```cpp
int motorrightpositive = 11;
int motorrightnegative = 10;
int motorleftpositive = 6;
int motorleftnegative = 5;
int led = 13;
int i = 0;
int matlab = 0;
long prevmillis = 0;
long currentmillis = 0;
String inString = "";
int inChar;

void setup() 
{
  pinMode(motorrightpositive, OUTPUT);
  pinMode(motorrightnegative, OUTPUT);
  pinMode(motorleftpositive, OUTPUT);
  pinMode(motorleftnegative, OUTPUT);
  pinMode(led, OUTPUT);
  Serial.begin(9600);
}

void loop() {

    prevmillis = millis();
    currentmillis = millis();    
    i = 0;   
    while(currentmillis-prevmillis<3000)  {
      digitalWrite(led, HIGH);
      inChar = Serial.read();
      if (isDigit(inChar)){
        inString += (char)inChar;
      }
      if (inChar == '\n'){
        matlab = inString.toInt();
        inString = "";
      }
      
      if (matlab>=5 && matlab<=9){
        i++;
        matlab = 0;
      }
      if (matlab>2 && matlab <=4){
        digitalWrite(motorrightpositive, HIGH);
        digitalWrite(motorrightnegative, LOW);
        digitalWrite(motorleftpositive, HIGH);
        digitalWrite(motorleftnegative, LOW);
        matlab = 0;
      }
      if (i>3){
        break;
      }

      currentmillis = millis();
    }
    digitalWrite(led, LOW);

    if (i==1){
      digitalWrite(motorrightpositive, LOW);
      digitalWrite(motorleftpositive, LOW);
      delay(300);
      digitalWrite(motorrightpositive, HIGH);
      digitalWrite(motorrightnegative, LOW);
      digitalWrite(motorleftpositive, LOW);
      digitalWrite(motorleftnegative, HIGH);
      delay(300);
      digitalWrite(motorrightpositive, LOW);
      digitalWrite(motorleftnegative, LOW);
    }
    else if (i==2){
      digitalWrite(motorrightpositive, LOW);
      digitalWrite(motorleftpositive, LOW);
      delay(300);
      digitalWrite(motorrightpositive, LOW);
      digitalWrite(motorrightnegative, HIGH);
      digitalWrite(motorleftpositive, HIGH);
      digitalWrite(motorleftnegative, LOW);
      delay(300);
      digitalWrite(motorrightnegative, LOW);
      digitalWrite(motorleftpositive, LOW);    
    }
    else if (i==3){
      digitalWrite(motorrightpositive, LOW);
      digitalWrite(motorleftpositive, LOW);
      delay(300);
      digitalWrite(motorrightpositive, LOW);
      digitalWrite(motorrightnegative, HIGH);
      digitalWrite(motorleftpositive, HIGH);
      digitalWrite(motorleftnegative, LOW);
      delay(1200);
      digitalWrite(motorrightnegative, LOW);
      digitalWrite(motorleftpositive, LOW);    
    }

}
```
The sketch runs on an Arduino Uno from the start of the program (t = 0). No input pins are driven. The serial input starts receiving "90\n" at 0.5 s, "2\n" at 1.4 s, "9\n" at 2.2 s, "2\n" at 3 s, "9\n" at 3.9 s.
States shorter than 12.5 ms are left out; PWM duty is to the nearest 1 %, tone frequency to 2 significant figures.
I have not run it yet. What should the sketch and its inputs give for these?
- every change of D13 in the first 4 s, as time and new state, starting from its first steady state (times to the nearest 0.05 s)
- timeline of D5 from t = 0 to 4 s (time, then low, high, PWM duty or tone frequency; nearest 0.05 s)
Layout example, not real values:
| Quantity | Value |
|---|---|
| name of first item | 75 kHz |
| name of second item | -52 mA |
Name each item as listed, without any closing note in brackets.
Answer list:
| Quantity | Value |
|---|---|
| every change of D13 in the first 4 s, as time and new state, starting from its first steady state | 0 s high; 3 s low; 3.6 s high |
| timeline of D5 from t = 0 to 4 s | 0 s low; 3.3 s high; 3.6 s low |
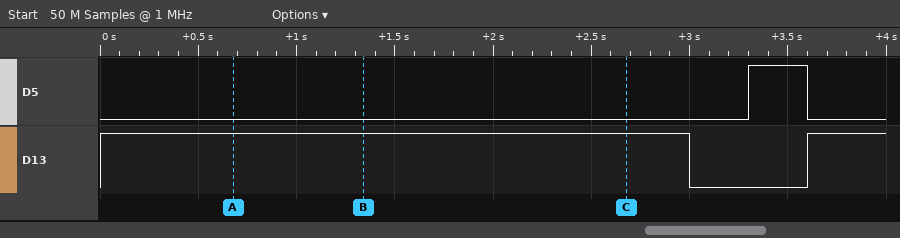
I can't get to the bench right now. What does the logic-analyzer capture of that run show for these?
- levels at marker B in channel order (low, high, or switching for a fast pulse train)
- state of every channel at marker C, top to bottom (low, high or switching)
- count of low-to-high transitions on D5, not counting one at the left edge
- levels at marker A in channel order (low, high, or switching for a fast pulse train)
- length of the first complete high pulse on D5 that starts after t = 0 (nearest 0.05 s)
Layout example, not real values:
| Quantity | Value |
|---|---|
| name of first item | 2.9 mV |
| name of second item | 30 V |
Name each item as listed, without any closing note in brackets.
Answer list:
| Quantity | Value |
|---|---|
| levels at marker B in channel order | D5 low, D13 high |
| state of every channel at marker C, top to bottom | D5 low, D13 high |
| count of low-to-high transitions on D5, not counting one at the left edge | 1 |
| levels at marker A in channel order | D5 low, D13 high |
| length of the first complete high pulse on D5 that starts after t = 0 | 0.30 s |
